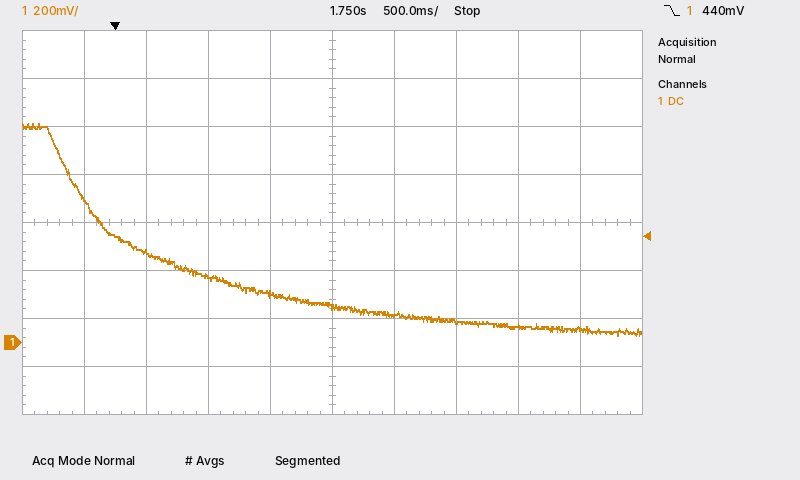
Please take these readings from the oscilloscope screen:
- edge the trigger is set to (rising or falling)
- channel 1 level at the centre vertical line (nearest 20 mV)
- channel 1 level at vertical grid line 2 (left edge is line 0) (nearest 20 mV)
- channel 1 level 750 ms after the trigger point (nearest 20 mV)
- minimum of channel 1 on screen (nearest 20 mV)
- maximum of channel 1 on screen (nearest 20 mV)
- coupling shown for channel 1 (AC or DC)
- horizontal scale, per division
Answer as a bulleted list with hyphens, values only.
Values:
- falling
- 160 mV
- 380 mV
- 280 mV
- 20 mV
- 920 mV
- DC
- 500 ms
